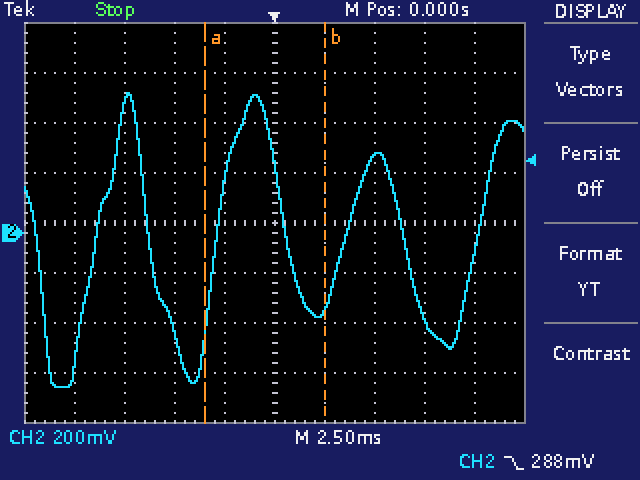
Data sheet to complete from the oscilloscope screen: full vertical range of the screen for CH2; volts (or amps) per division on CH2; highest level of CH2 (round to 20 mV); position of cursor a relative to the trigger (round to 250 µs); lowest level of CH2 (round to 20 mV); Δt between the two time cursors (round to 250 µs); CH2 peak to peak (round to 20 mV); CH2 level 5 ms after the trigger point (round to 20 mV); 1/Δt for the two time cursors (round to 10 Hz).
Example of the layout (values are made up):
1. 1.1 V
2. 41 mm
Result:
1. 1.6 V
2. 200 mV
3. 560 mV
4. -3.50 ms
5. -620 mV
6. 6.00 ms
7. 1.18 V
8. 300 mV
9. 170 Hz
